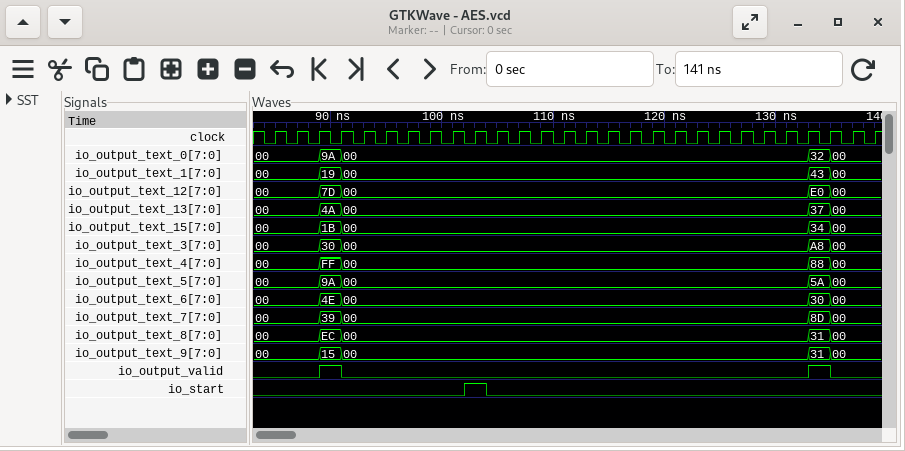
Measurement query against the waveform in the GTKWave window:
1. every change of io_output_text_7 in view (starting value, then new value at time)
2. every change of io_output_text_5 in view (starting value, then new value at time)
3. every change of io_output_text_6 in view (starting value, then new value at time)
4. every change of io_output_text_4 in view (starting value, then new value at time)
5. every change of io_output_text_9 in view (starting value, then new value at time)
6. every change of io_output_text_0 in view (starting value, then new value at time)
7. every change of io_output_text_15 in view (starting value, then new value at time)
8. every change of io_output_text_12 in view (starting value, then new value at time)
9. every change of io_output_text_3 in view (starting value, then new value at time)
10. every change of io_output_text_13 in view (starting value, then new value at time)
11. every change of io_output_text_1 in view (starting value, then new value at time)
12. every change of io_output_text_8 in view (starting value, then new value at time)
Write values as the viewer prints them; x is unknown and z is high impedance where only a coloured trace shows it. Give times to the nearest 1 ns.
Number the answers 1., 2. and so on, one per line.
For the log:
1. 00, 39 at 89 ns, 00 at 91 ns, 8D at 133 ns, 00 at 135 ns
2. 00, 9A at 89 ns, 00 at 91 ns, 5A at 133 ns, 00 at 135 ns
3. 00, 4E at 89 ns, 00 at 91 ns, 30 at 133 ns, 00 at 135 ns
4. 00, FF at 89 ns, 00 at 91 ns, 88 at 133 ns, 00 at 135 ns
5. 00, 15 at 89 ns, 00 at 91 ns, 31 at 133 ns, 00 at 135 ns
6. 00, 9A at 89 ns, 00 at 91 ns, 32 at 133 ns, 00 at 135 ns
7. 00, 1B at 89 ns, 00 at 91 ns, 34 at 133 ns, 00 at 135 ns
8. 00, 7D at 89 ns, 00 at 91 ns, E0 at 133 ns, 00 at 135 ns
9. 00, 30 at 89 ns, 00 at 91 ns, A8 at 133 ns, 00 at 135 ns
10. 00, 4A at 89 ns, 00 at 91 ns, 37 at 133 ns, 00 at 135 ns
11. 00, 19 at 89 ns, 00 at 91 ns, 43 at 133 ns, 00 at 135 ns
12. 00, EC at 89 ns, 00 at 91 ns, 31 at 133 ns, 00 at 135 ns
